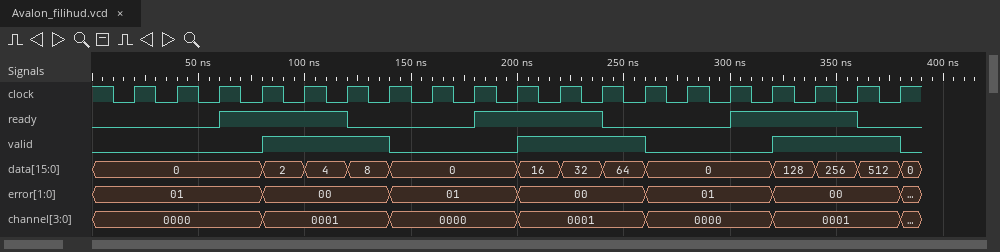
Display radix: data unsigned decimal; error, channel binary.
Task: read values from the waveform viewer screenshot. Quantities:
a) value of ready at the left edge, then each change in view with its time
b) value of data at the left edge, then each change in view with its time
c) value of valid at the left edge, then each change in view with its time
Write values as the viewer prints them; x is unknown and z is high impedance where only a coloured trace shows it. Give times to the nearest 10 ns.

0, 1 at 60 ns, 0 at 120 ns, 1 at 180 ns, 0 at 240 ns, 1 at 300 ns, 0 at 360 ns
0, 2 at 80 ns, 4 at 100 ns, 8 at 120 ns, 0 at 140 ns, 16 at 200 ns, 32 at 220 ns, 64 at 240 ns, 0 at 260 ns, 128 at 320 ns, 256 at 340 ns, 512 at 360 ns, 0 at 380 ns
0, 1 at 80 ns, 0 at 140 ns, 1 at 200 ns, 0 at 260 ns, 1 at 320 ns, 0 at 380 ns
